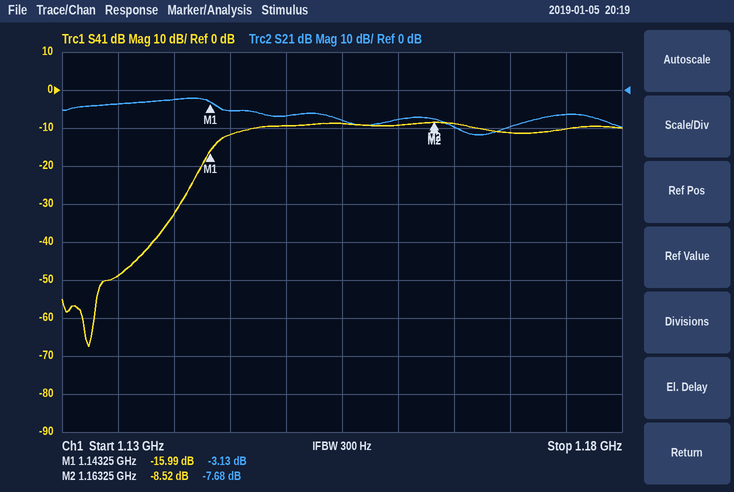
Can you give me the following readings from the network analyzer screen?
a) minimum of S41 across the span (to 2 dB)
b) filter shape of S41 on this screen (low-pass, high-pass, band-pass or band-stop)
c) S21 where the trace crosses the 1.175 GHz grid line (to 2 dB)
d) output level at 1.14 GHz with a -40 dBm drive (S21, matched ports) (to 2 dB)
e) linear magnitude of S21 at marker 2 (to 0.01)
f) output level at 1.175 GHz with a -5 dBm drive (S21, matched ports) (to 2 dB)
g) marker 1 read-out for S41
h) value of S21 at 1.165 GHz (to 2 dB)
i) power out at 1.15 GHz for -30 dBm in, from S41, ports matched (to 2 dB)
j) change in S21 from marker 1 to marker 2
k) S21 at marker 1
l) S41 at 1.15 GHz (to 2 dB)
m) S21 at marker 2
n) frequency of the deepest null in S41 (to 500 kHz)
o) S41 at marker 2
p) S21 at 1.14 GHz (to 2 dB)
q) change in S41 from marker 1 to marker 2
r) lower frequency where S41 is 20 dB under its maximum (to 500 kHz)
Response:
-68 dB
high-pass
-6 dB
-42 dBm
0.41
-12 dBm
-15.99 dB
-10 dB
-40 dBm
-4.55 dB
-3.13 dB
-10 dB
-7.68 dB
1.1325 GHz
-8.52 dB
-2 dB
7.47 dB
1.1410 GHz
